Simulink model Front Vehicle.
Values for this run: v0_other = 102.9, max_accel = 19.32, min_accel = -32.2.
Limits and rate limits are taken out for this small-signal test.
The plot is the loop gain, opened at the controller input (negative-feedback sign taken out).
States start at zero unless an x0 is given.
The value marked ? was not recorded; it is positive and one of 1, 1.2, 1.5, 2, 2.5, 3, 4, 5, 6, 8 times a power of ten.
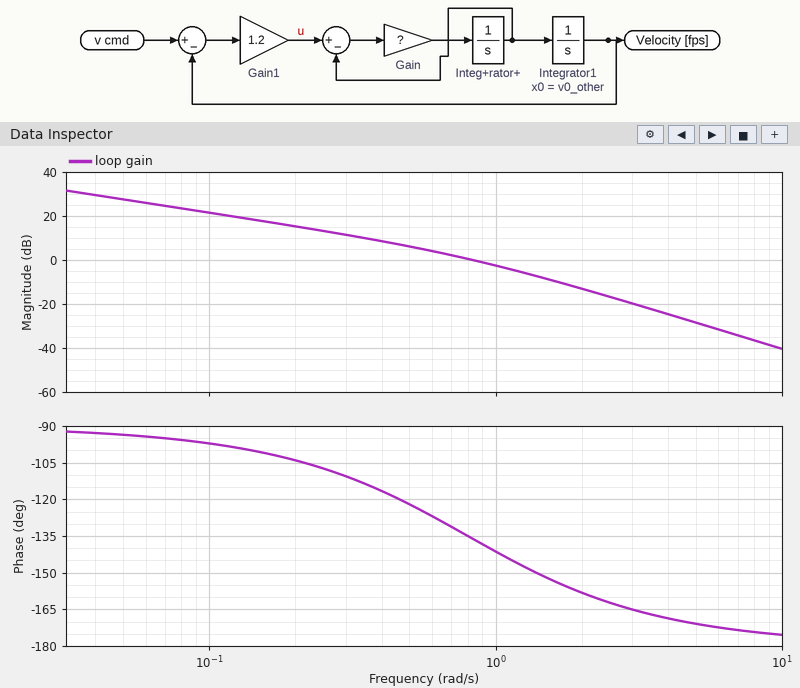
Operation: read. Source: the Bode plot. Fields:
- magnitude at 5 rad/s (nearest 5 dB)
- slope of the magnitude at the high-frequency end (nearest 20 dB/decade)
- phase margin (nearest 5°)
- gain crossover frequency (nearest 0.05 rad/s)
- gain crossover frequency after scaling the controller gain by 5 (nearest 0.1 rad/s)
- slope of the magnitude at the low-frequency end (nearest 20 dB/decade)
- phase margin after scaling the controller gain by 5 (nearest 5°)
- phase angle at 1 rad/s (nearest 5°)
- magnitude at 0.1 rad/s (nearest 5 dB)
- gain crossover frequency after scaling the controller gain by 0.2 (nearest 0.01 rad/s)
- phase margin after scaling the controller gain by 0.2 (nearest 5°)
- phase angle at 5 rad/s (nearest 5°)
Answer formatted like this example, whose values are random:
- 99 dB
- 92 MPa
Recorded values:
- -30 dB
- -40 dB/decade
- 45°
- 0.85 rad/s
- 2.1 rad/s
- -20 dB/decade
- 20°
- -140°
- 20 dB
- 0.23 rad/s
- 75°
- -170°
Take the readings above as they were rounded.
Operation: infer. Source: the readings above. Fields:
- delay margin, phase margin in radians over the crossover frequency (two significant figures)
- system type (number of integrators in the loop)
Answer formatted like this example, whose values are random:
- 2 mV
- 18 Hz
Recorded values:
- 0.92 s
- 1
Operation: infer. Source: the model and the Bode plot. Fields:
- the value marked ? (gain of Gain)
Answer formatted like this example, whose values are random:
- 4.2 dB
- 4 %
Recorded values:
- 0.8
